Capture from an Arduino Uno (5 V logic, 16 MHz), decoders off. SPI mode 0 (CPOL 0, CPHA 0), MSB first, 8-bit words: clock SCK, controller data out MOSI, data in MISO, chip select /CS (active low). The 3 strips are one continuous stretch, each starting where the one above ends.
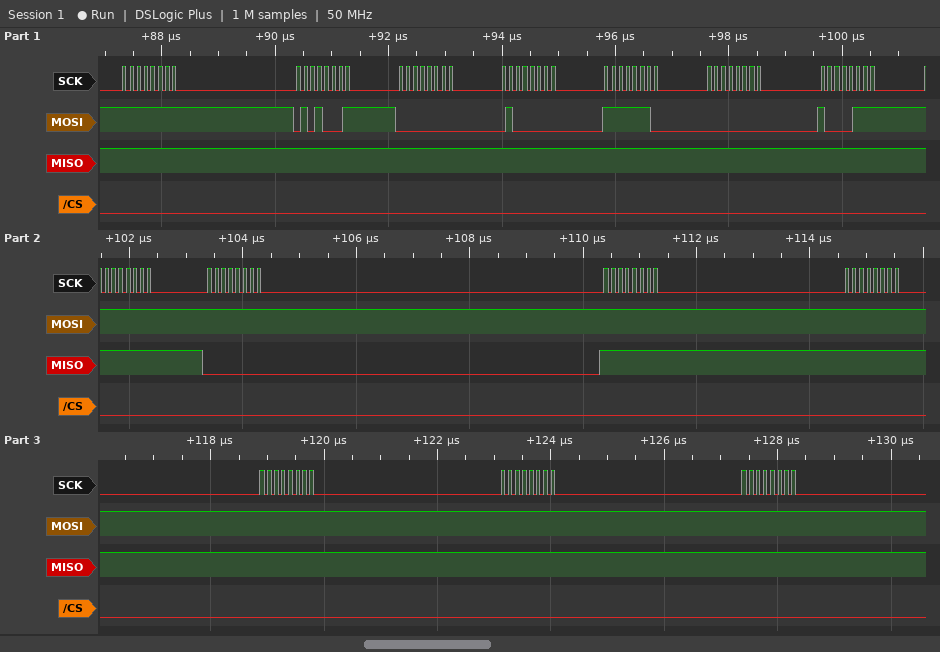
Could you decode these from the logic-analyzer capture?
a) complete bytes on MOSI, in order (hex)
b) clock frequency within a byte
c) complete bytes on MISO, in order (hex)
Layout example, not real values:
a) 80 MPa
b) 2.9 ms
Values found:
a) FF 51 00 40 FE 00 87 FF FF FF FF FF FF FF
b) 8 MHz
c) FF FF FF FF FF FF FF FF 00 FF FF FF FF FF
